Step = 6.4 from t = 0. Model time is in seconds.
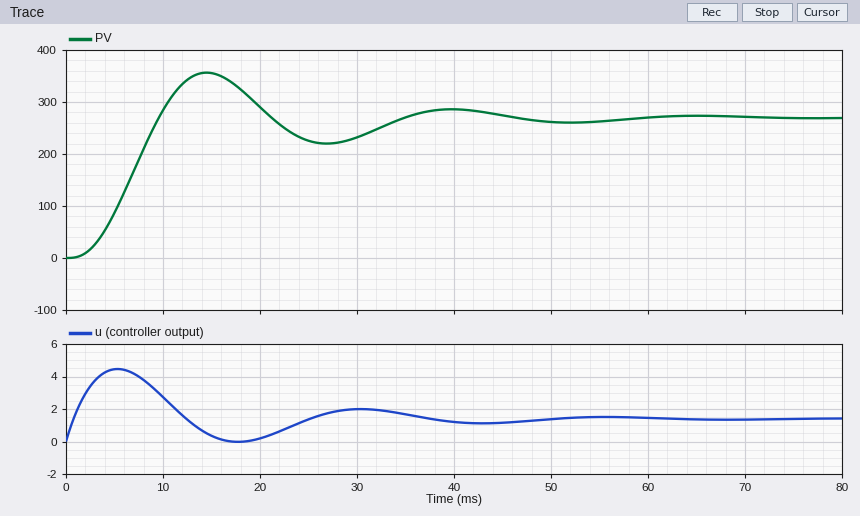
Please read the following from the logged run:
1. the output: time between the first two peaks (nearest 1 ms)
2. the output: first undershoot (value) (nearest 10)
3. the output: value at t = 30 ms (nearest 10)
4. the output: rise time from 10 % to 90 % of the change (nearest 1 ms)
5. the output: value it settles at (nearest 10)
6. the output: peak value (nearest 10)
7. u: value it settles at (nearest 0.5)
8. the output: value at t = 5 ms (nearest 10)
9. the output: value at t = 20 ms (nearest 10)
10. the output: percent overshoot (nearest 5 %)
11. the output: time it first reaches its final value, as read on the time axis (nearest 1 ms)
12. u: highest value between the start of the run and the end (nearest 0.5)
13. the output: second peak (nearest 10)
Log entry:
25 ms
220
230
6 ms
270
360
1.5
90
290
30 %
10 ms
4.5
290
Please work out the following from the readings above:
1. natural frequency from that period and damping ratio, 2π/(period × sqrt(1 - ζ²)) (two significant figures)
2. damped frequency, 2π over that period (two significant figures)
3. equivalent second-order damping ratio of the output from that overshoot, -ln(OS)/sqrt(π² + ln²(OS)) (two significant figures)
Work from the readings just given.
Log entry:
0.27 rad/ms
0.25 rad/ms
0.36
